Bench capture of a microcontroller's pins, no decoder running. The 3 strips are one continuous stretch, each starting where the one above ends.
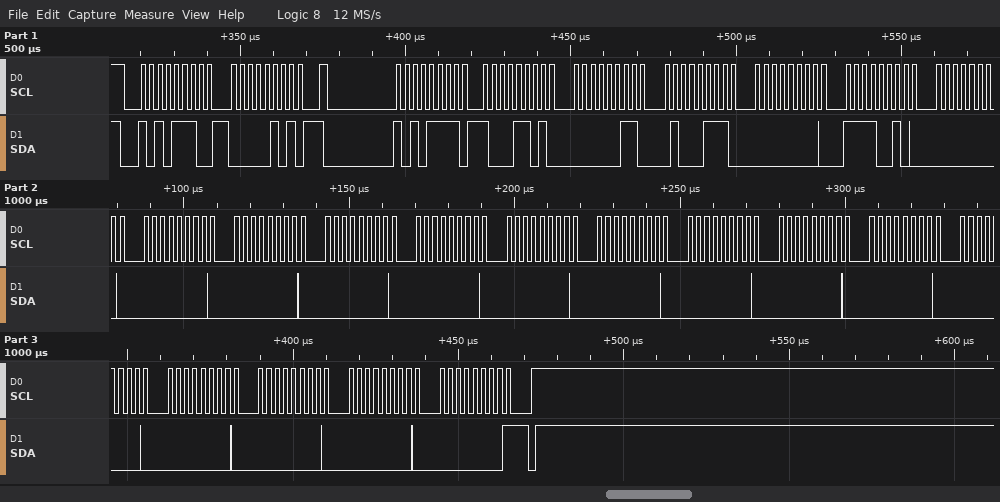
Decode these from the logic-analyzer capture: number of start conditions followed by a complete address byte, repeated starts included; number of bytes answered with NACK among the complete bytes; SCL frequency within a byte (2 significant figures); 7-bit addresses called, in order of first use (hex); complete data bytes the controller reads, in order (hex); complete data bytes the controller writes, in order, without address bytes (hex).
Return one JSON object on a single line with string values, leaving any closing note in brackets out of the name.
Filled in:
{"number of start conditions followed by a complete address byte, repeated starts included": "2", "number of bytes answered with NACK among the complete bytes": "1", "SCL frequency within a byte": "400 kHz", "7-bit addresses called, in order of first use": "0x57", "complete data bytes the controller reads, in order": "8D 03 47 00 F2 00 00 00 00 00 00 00 00 00 00 00 00 00 00 00", "complete data bytes the controller writes, in order, without address bytes": "05"}
